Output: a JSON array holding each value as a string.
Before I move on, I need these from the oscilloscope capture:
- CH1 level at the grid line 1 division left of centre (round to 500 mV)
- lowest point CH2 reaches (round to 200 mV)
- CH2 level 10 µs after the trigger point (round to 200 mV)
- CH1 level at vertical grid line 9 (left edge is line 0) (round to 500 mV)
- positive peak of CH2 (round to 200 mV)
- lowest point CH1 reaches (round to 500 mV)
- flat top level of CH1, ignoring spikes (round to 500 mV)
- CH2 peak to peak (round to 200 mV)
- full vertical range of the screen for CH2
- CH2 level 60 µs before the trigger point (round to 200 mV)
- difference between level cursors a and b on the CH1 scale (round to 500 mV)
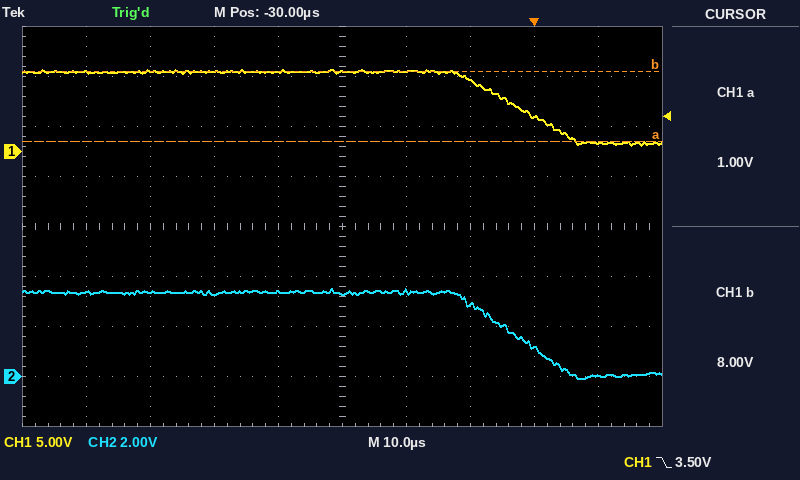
["8.0 V", "0.0 V", "0.0 V", "1.0 V", "3.6 V", "500 mV", "8.0 V", "3.6 V", "16 V", "3.4 V", "7.0 V"]
